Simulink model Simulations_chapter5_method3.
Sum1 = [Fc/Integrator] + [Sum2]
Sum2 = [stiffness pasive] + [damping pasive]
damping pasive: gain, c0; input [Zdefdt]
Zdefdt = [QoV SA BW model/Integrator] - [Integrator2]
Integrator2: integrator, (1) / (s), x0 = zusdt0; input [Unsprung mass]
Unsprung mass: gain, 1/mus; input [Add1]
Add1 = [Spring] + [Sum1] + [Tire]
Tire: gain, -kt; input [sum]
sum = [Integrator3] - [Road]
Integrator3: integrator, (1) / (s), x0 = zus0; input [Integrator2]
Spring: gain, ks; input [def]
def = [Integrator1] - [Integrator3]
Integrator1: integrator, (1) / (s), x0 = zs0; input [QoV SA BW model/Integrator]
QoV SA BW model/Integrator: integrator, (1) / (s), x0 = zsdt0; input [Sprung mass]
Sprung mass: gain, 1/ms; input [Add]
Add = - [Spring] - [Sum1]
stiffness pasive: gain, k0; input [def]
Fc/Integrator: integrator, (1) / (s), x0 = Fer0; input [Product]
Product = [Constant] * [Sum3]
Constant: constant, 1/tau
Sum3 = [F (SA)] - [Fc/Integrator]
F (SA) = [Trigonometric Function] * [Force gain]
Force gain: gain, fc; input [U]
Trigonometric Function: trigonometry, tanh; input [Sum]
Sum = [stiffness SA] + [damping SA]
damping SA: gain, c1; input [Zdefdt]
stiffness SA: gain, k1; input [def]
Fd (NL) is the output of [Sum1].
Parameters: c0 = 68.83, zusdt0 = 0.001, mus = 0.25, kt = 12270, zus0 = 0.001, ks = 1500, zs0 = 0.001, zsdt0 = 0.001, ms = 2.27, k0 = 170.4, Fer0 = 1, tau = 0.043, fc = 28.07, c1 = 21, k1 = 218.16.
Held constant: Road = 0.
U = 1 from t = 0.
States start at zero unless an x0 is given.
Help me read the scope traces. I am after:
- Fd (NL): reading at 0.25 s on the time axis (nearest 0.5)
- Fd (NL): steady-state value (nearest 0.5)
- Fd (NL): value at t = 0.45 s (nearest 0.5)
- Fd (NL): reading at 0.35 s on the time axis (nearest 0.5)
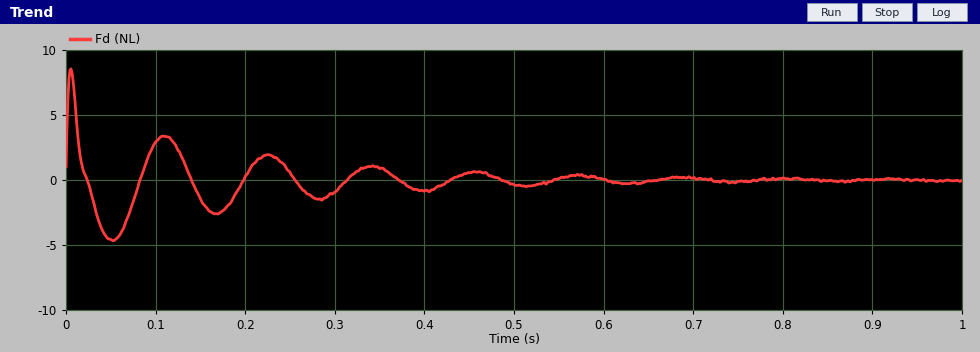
0.5
0.0
0.5
1.0
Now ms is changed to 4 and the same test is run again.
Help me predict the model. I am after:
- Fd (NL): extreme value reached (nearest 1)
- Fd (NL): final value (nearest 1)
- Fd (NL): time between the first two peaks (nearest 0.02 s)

9
0
0.14 s
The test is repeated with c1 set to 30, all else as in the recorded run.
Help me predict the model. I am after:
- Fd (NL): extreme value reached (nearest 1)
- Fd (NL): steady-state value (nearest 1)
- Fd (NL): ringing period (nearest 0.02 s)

9
0
0.10 s
